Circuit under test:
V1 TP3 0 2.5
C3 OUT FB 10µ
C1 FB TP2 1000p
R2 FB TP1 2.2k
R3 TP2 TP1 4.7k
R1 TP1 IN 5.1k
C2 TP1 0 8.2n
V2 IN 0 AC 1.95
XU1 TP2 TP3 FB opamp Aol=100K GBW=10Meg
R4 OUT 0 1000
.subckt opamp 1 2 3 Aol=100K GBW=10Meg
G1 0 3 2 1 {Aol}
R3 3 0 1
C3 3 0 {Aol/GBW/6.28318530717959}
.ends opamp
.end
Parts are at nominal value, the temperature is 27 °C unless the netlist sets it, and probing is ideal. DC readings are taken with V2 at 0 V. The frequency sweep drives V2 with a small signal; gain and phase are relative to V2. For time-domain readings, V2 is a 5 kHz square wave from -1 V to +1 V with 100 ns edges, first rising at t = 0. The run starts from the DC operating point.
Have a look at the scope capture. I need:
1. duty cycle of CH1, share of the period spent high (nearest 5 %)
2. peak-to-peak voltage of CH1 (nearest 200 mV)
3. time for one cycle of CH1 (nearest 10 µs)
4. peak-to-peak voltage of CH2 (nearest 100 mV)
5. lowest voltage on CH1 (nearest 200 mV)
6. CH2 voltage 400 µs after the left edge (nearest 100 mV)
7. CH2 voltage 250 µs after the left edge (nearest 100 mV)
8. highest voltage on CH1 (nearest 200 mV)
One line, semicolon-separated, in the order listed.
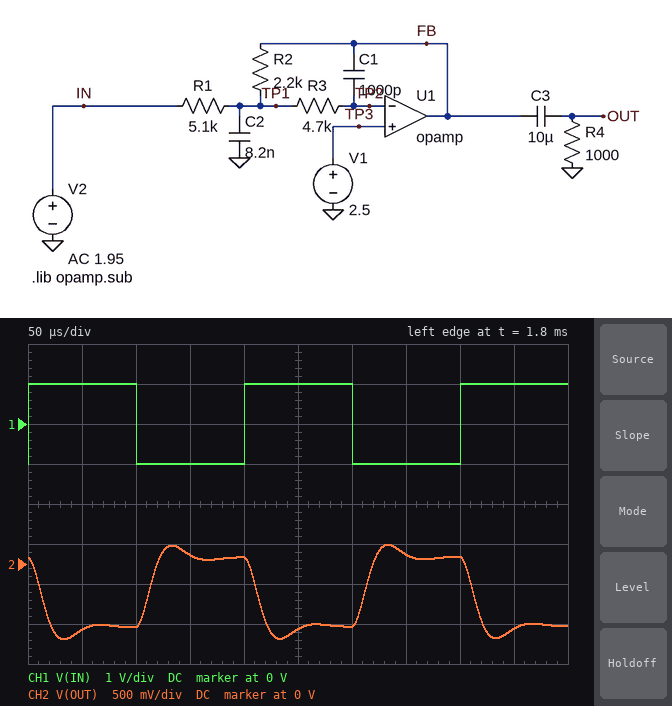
50 %; 2.0 V; 200 µs; 1.2 V; -1.0 V; 100 mV; -800 mV; 1.0 V
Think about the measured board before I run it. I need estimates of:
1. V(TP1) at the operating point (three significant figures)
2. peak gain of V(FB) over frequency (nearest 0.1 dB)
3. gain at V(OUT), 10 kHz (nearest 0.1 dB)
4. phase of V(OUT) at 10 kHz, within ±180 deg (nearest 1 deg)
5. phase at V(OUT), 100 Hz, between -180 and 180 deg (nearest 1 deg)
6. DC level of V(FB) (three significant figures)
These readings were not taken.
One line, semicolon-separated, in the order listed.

2.50 V; -5.9 dB; -6.1 dB; 140 deg; -171 deg; 3.58 V
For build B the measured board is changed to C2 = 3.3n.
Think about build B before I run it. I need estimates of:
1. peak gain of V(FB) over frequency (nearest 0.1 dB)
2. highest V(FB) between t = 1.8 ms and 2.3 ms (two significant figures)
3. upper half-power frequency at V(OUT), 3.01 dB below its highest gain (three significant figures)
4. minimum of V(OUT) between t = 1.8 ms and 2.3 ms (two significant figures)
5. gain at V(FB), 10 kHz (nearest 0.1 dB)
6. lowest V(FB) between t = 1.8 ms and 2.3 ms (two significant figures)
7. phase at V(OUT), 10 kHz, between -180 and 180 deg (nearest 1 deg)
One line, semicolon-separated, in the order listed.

-7.3 dB; 4.0 V; 25.1 kHz; -810 mV; -7.6 dB; 3.1 V; 147 deg
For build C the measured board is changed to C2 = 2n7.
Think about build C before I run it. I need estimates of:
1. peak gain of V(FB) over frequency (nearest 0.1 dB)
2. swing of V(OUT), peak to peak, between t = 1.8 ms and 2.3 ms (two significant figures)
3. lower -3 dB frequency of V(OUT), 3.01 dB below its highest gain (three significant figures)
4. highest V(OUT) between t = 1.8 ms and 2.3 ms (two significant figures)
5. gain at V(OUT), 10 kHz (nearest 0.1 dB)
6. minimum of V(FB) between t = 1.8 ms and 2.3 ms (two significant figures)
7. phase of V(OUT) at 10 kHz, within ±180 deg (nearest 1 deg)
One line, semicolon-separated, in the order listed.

-7.3 dB; 890 mV; 15.9 Hz; 92 mV; -7.7 dB; 3.1 V; 148 deg
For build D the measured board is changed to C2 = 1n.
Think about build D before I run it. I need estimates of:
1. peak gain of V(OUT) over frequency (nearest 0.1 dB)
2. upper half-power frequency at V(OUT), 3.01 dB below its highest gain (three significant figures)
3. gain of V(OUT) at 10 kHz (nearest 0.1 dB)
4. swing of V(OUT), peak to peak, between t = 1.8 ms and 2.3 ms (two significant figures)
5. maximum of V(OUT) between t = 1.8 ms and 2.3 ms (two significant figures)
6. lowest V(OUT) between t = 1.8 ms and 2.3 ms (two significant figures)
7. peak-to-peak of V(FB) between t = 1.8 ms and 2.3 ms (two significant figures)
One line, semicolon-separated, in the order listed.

-7.3 dB; 20.4 kHz; -8.2 dB; 870 mV; 85 mV; -790 mV; 860 mV
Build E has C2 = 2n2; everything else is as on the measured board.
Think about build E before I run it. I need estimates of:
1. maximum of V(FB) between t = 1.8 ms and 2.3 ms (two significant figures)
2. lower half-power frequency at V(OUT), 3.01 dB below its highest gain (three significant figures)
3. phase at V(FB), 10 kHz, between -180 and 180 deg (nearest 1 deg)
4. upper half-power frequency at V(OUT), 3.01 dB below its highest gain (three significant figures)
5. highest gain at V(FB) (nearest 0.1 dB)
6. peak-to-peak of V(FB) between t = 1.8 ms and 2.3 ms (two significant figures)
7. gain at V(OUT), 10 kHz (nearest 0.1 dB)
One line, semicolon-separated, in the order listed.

4.0 V; 15.9 Hz; 148 deg; 23.6 kHz; -7.3 dB; 860 mV; -7.9 dB
